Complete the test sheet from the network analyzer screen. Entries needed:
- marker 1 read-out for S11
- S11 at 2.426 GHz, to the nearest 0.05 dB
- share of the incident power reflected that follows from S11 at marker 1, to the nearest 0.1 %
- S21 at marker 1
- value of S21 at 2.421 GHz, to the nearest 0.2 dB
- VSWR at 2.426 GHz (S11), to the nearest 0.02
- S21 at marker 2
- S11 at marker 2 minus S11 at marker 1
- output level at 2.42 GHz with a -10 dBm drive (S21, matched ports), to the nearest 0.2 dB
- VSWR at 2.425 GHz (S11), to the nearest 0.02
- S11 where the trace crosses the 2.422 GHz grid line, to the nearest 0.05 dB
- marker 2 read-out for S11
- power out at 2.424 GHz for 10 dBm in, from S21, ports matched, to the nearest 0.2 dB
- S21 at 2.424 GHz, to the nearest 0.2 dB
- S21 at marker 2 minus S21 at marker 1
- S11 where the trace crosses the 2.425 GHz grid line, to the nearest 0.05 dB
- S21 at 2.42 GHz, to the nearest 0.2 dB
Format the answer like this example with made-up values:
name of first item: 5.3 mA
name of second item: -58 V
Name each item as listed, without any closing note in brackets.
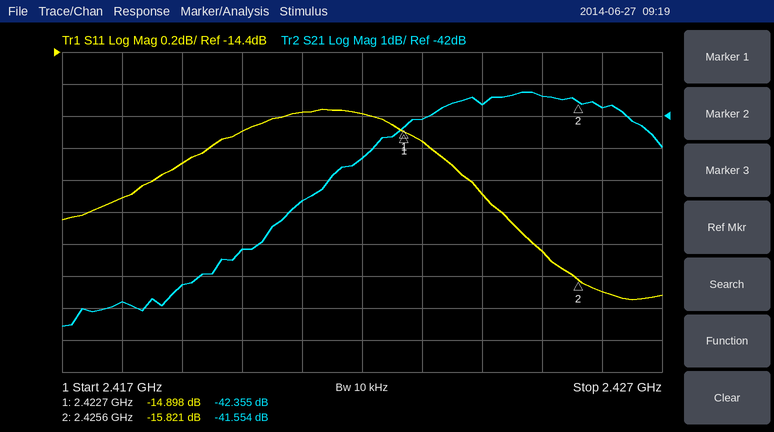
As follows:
marker 1 read-out for S11: -14.898 dB
S11 at 2.426 GHz, to the nearest 0.05 dB: -15.90 dB
share of the incident power reflected that follows from S11 at marker 1, to the nearest 0.1 %: 3.2 %
S21 at marker 1: -42.355 dB
value of S21 at 2.421 GHz, to the nearest 0.2 dB: -44.6 dB
VSWR at 2.426 GHz (S11), to the nearest 0.02: 1.38
S21 at marker 2: -41.554 dB
S11 at marker 2 minus S11 at marker 1: -0.923 dB
output level at 2.42 GHz with a -10 dBm drive (S21, matched ports), to the nearest 0.2 dB: -56.2 dBm
VSWR at 2.425 GHz (S11), to the nearest 0.02: 1.40
S11 where the trace crosses the 2.422 GHz grid line, to the nearest 0.05 dB: -14.80 dB
marker 2 read-out for S11: -15.821 dB
power out at 2.424 GHz for 10 dBm in, from S21, ports matched, to the nearest 0.2 dB: -31.6 dBm
S21 at 2.424 GHz, to the nearest 0.2 dB: -41.6 dB
S21 at marker 2 minus S21 at marker 1: 0.801 dB
S11 where the trace crosses the 2.425 GHz grid line, to the nearest 0.05 dB: -15.65 dB
S21 at 2.42 GHz, to the nearest 0.2 dB: -46.2 dB
